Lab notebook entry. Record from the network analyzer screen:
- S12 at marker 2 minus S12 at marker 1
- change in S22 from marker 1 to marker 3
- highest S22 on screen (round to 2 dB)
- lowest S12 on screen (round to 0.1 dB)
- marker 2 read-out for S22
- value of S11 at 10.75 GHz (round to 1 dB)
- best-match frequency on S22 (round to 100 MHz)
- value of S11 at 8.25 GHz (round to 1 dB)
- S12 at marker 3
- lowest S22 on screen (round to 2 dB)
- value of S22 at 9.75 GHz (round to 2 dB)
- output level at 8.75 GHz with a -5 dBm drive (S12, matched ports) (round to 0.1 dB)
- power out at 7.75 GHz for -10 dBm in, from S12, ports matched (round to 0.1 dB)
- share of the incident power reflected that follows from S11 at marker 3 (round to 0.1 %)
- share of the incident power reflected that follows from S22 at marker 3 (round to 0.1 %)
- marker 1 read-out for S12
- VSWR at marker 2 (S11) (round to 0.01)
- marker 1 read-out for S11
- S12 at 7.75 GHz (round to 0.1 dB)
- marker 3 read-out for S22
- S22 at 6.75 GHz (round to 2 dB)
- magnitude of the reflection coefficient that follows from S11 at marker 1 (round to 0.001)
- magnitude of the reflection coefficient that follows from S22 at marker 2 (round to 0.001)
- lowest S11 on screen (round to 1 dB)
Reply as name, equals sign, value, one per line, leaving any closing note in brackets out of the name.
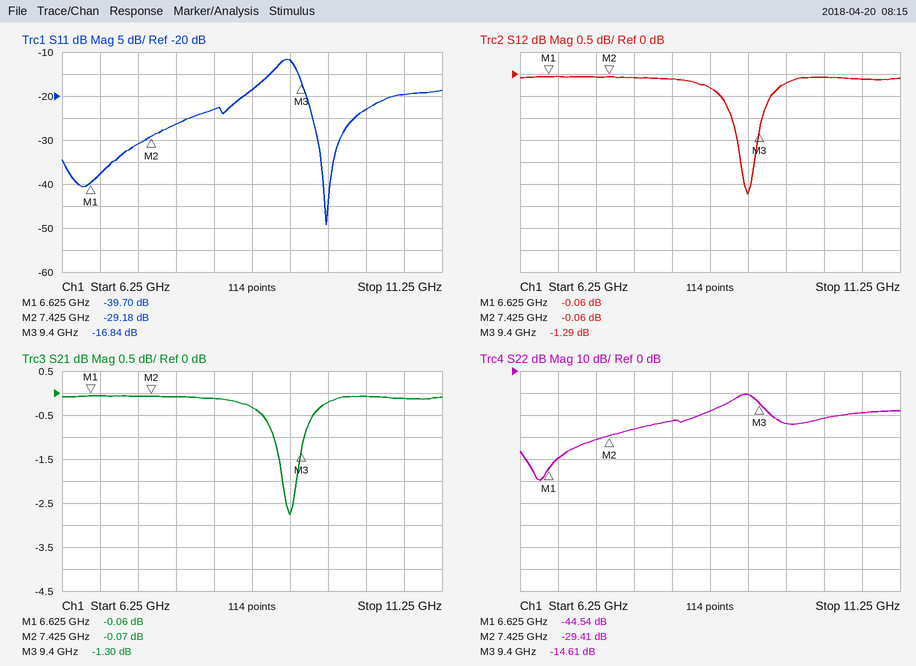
S12 at marker 2 minus S12 at marker 1 = 0.00 dB
change in S22 from marker 1 to marker 3 = 29.93 dB
highest S22 on screen = -10 dB
lowest S12 on screen = -2.7 dB
marker 2 read-out for S22 = -29.41 dB
value of S11 at 10.75 GHz = -20 dB
best-match frequency on S22 = 6.5 GHz
value of S11 at 8.25 GHz = -23 dB
S12 at marker 3 = -1.29 dB
lowest S22 on screen = -50 dB
value of S22 at 9.75 GHz = -24 dB
output level at 8.75 GHz with a -5 dBm drive (S12, matched ports) = -5.3 dBm
power out at 7.75 GHz for -10 dBm in, from S12, ports matched = -10.1 dBm
share of the incident power reflected that follows from S11 at marker 3 = 2.1 %
share of the incident power reflected that follows from S22 at marker 3 = 3.5 %
marker 1 read-out for S12 = -0.06 dB
VSWR at marker 2 (S11) = 1.07
marker 1 read-out for S11 = -39.70 dB
S12 at 7.75 GHz = -0.1 dB
marker 3 read-out for S22 = -14.61 dB
S22 at 6.75 GHz = -40 dB
magnitude of the reflection coefficient that follows from S11 at marker 1 = 0.010
magnitude of the reflection coefficient that follows from S22 at marker 2 = 0.034
lowest S11 on screen = -49 dB
